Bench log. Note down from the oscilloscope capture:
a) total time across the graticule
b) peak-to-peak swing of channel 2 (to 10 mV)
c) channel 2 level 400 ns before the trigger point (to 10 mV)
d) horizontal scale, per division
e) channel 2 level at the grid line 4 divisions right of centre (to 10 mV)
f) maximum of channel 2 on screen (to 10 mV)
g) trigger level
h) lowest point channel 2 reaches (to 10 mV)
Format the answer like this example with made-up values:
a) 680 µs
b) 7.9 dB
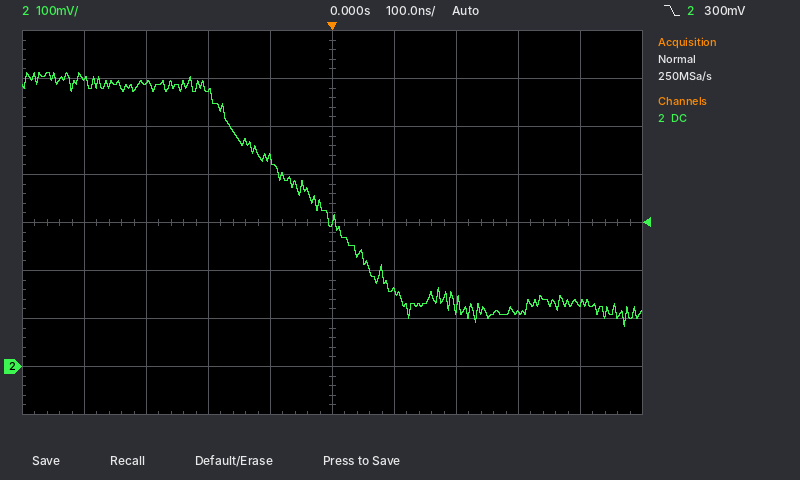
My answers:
a) 1 µs
b) 530 mV
c) 600 mV
d) 100 ns
e) 130 mV
f) 610 mV
g) 300 mV
h) 80 mV
